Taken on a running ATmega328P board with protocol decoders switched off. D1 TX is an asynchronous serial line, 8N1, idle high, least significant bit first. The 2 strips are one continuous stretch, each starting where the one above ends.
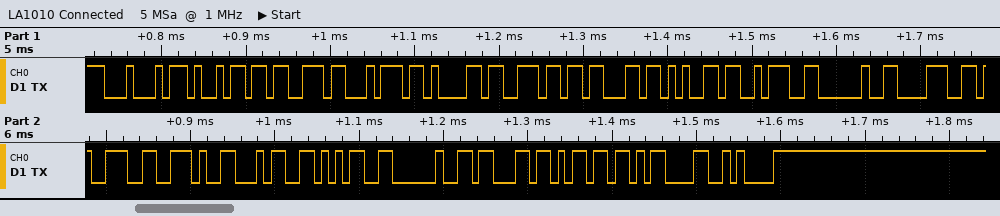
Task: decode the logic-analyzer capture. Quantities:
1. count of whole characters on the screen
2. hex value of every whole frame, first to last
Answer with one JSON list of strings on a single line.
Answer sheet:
["20", "44 69 73 74 61 6E 63 65 3A 20 38 39 2E 34 35 20 63 6D 0D 0A"]
